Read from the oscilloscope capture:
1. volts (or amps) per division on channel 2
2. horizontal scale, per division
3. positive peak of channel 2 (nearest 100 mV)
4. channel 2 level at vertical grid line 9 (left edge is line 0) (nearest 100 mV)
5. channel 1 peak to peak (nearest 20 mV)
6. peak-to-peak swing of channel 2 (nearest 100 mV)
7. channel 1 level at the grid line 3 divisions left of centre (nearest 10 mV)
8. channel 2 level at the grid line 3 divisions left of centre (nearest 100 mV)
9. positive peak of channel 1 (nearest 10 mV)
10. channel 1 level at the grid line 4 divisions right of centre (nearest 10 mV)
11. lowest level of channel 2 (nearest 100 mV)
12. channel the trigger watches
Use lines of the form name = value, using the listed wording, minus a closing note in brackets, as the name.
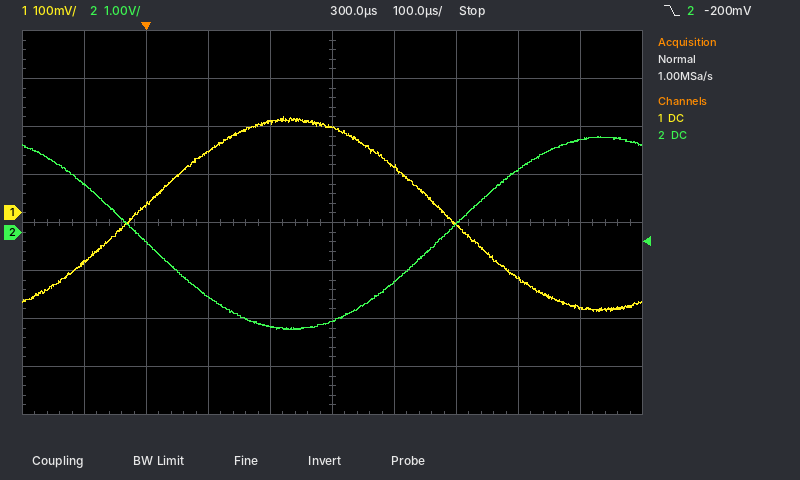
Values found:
volts (or amps) per division on channel 2 = 1 V
horizontal scale, per division = 100 µs
positive peak of channel 2 = 2.0 V
channel 2 level at vertical grid line 9 (left edge is line 0) = 1.9 V
channel 1 peak to peak = 400 mV
peak-to-peak swing of channel 2 = 4.0 V
channel 1 level at the grid line 3 divisions left of centre = 20 mV
channel 2 level at the grid line 3 divisions left of centre = -200 mV
positive peak of channel 1 = 200 mV
channel 1 level at the grid line 4 divisions right of centre = -200 mV
lowest level of channel 2 = -2.0 V
channel the trigger watches = channel 2
